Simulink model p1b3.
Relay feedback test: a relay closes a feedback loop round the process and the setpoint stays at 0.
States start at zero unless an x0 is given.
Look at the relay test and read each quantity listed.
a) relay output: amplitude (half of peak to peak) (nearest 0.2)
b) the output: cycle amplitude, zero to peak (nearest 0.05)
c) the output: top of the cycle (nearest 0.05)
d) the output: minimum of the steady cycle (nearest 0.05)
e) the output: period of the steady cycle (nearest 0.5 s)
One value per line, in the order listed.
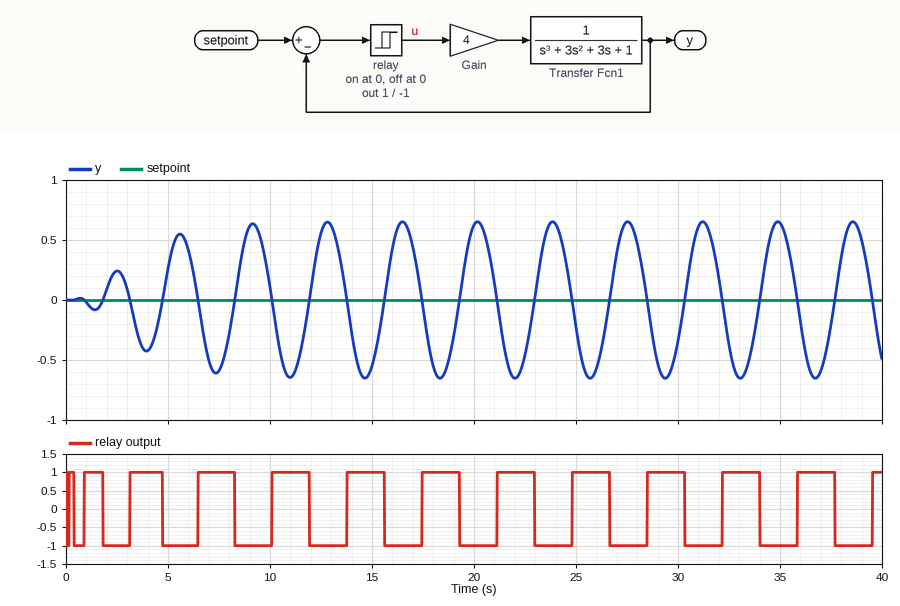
1.0
0.65
0.65
-0.65
3.5 s
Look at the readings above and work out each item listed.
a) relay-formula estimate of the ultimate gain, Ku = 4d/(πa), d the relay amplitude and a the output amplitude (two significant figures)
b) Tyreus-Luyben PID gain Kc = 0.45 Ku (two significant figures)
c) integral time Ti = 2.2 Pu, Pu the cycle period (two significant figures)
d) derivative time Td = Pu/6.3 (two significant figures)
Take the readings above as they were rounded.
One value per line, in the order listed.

2.0
0.90
7.7 s
0.56 s
